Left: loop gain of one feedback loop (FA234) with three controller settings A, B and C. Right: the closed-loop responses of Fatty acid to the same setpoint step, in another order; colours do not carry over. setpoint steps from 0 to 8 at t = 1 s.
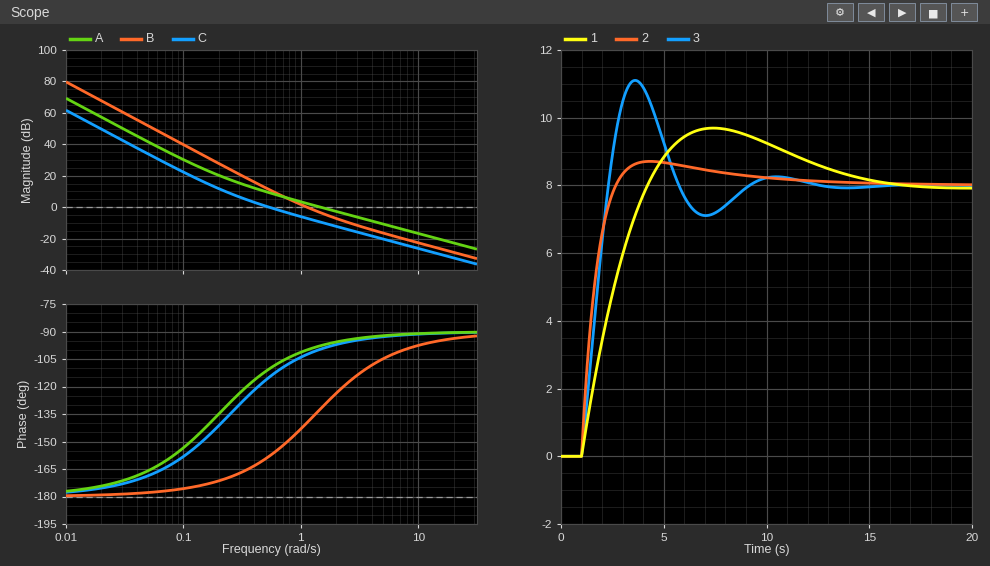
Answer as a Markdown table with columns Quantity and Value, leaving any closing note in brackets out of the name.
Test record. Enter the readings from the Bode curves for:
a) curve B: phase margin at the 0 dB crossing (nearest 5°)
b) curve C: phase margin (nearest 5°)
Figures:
| Quantity | Value |
|---|---|
| curve B: phase margin at the 0 dB crossing | 40° |
| curve C: phase margin | 65° |
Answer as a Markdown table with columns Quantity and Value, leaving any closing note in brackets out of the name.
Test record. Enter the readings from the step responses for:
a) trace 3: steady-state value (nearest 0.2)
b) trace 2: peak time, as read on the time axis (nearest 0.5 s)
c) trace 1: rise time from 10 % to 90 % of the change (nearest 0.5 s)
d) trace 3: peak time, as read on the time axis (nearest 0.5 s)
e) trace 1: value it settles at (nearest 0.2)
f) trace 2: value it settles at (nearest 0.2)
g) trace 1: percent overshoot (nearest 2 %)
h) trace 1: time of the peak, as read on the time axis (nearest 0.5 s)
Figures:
| Quantity | Value |
|---|---|
| trace 3: steady-state value | 8.0 |
| trace 2: peak time, as read on the time axis | 4.5 s |
| trace 1: rise time from 10 % to 90 % of the change | 2.5 s |
| trace 3: peak time, as read on the time axis | 3.5 s |
| trace 1: value it settles at | 8.0 |
| trace 2: value it settles at | 8.0 |
| trace 1: percent overshoot | 22 % |
| trace 1: time of the peak, as read on the time axis | 7.5 s |
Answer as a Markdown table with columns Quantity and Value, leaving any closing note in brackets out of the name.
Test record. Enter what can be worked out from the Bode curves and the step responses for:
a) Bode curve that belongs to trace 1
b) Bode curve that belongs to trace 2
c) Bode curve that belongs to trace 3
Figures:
| Quantity | Value |
|---|---|
| Bode curve that belongs to trace 1 | C |
| Bode curve that belongs to trace 2 | A |
| Bode curve that belongs to trace 3 | B |
